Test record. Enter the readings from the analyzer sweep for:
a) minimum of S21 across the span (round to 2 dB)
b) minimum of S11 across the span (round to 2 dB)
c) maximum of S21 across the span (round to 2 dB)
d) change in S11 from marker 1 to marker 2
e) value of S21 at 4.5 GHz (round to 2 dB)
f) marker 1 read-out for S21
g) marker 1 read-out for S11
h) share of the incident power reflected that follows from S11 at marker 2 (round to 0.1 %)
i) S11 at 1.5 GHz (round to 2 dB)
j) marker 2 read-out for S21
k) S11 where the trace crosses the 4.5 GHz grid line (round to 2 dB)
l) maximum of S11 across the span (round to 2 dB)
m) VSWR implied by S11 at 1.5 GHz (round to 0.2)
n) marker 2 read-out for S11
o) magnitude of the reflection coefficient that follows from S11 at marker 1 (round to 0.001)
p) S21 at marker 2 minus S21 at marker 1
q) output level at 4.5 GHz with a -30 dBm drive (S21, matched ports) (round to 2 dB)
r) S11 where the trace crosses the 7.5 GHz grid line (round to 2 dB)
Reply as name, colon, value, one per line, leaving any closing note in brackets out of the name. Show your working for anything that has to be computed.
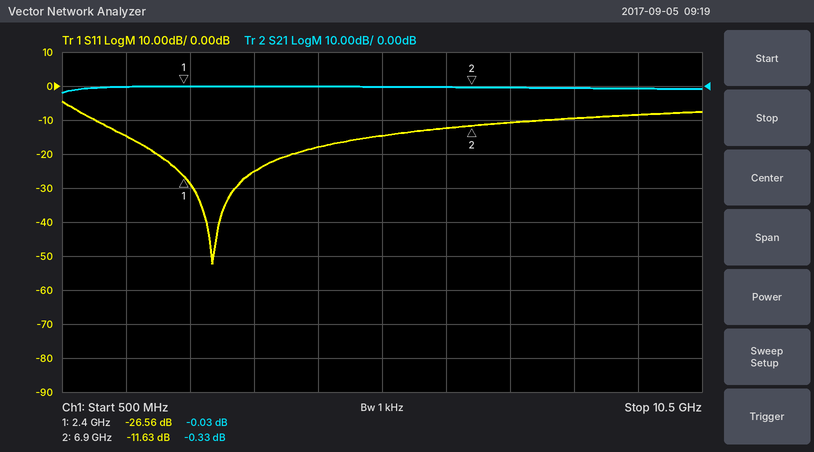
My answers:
minimum of S21 across the span: -2 dB
minimum of S11 across the span: -52 dB
maximum of S21 across the span: 0 dB
change in S11 from marker 1 to marker 2: -11.63 − (-26.56) = 14.93 dB
value of S21 at 4.5 GHz: 0 dB
marker 1 read-out for S21: -0.03 dB
marker 1 read-out for S11: -26.56 dB
share of the incident power reflected that follows from S11 at marker 2: 10^(-11.63/10) ≈ 6.9 %
S11 at 1.5 GHz: -14 dB
marker 2 read-out for S21: -0.33 dB
S11 where the trace crosses the 4.5 GHz grid line: -18 dB
maximum of S11 across the span: -4 dB
VSWR implied by S11 at 1.5 GHz: |Γ| = 10^(-14/20) = 0.1995; VSWR = (1 + 0.1995)/(1 − 0.1995) ≈ 1.50, so 1.4 to the nearest 0.2
marker 2 read-out for S11: -11.63 dB
magnitude of the reflection coefficient that follows from S11 at marker 1: 10^(-26.56/20) ≈ 0.047
S21 at marker 2 minus S21 at marker 1: -0.33 − (-0.03) = -0.30 dB
output level at 4.5 GHz with a -30 dBm drive (S21, matched ports): -30 dBm + (0 dB) = -30 dBm
S11 where the trace crosses the 7.5 GHz grid line: -10 dB
